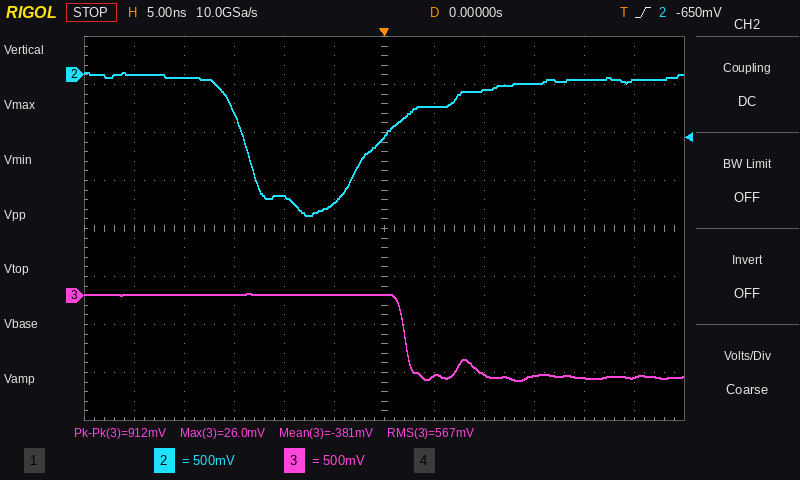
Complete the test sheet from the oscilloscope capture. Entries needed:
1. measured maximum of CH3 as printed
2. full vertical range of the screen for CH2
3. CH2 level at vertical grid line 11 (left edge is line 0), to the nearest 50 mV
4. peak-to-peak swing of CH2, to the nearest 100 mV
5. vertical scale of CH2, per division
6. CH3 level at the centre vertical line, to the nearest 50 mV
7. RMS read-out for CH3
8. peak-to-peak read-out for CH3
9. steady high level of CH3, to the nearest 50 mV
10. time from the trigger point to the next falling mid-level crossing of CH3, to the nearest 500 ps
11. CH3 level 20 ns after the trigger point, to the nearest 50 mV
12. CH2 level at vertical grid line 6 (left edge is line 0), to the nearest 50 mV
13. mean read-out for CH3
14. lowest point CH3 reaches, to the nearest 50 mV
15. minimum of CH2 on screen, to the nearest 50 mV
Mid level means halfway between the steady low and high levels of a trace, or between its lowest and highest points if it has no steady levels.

26.0 mV
4 V
-50 mV
1.50 V
500 mV
0 mV
567 mV
912 mV
0 mV
2.0 ns
-850 mV
-650 mV
-381 mV
-900 mV
-1.45 V
